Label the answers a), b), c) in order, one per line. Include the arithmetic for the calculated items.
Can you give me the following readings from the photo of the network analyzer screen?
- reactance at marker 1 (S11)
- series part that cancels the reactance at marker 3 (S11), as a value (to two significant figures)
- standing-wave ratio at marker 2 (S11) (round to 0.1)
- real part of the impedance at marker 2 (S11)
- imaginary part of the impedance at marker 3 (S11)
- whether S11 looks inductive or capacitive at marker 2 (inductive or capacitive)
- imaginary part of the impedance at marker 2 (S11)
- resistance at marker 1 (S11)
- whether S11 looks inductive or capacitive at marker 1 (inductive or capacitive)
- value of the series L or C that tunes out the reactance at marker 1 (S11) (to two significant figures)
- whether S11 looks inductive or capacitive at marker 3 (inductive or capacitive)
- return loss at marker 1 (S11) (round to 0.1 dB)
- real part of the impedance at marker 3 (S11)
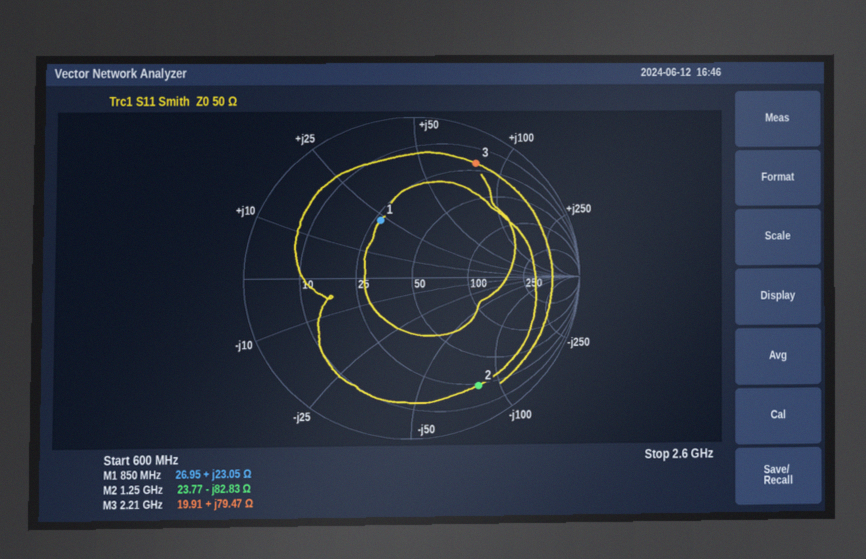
a) +23.05 Ω
b) C = 1/(2π × 2.21 GHz × 79.47 Ω) ≈ 906 fF, so 910 fF to two significant figures
c) 8.2
d) 23.77 Ω
e) +79.47 Ω
f) capacitive
g) -82.83 Ω
h) 26.95 Ω
i) inductive
j) C = 1/(2π × 850 MHz × 23.05 Ω) ≈ 8.1 pF
k) inductive
l) 7.8 dB
m) 19.91 Ω
